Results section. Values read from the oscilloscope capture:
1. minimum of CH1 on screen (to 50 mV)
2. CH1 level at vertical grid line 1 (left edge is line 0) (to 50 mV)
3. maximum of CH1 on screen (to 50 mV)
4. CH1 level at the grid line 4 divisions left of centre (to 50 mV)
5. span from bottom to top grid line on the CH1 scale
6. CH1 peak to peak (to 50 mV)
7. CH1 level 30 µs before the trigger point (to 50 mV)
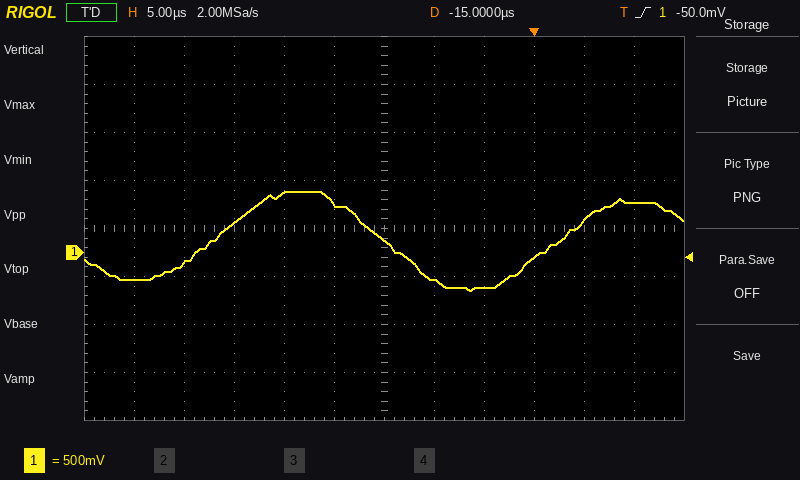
-400 mV
-300 mV
650 mV
-100 mV
4 V
1.05 V
300 mV
